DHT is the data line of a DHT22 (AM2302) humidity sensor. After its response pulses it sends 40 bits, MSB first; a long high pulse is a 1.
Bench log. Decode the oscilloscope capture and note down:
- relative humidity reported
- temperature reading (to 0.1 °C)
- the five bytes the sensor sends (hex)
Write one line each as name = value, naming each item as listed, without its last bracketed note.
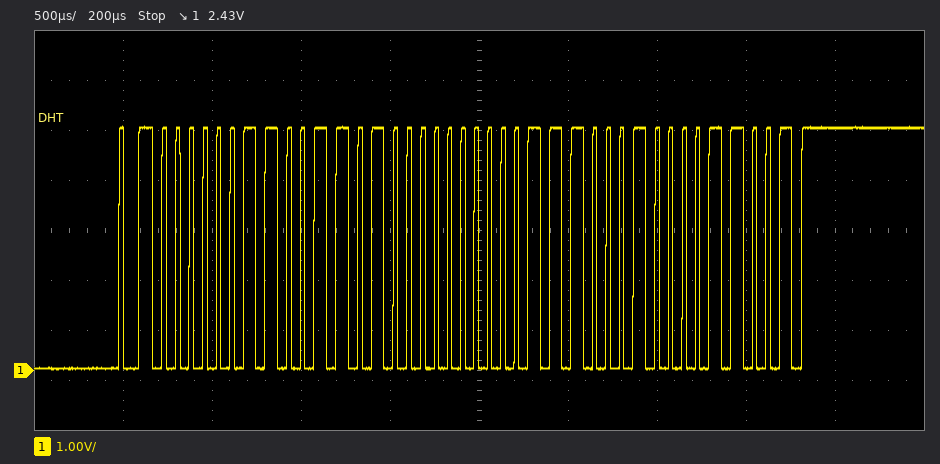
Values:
relative humidity reported = 82.0 %
temperature reading = 22.6 °C
the five bytes the sensor sends = 03 34 00 E2 19
